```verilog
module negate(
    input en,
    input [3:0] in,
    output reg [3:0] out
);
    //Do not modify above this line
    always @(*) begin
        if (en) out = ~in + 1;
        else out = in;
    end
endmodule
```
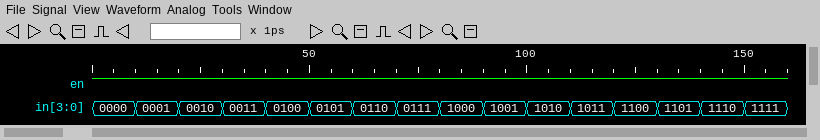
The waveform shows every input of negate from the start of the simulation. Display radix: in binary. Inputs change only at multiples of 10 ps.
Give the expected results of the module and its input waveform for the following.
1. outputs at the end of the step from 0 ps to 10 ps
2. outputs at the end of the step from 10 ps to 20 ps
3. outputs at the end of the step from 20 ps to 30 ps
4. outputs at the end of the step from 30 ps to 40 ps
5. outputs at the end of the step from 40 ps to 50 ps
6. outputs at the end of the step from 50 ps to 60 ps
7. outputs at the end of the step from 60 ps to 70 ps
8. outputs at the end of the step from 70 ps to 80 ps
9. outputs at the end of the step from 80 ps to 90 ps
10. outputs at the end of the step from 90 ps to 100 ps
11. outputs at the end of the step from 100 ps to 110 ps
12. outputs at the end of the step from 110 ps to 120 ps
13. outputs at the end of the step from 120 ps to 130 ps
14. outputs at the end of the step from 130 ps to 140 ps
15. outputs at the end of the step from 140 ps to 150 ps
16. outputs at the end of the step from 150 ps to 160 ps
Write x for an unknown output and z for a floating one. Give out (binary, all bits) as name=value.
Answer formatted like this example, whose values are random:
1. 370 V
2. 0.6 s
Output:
1. out=0000
2. out=1111
3. out=1110
4. out=1101
5. out=1100
6. out=1011
7. out=1010
8. out=1001
9. out=1000
10. out=0111
11. out=0110
12. out=0101
13. out=0100
14. out=0011
15. out=0010
16. out=0001
